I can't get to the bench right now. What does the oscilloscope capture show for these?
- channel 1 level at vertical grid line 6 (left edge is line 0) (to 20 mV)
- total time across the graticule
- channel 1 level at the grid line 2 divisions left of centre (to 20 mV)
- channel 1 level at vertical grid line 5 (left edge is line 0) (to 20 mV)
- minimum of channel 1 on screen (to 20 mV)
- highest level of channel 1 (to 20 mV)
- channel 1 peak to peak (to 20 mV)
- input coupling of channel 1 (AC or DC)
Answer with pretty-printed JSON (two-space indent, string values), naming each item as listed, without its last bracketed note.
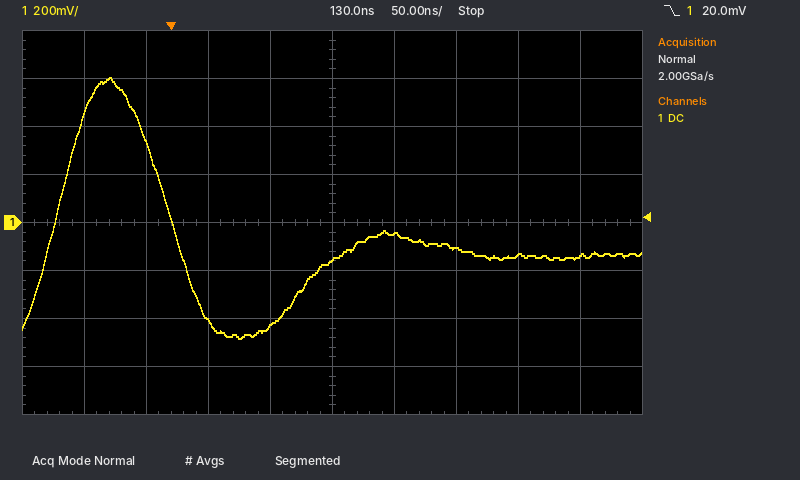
{
  "channel 1 level at vertical grid line 6 (left edge is line 0)": "-40 mV",
  "total time across the graticule": "500 ns",
  "channel 1 level at the grid line 2 divisions left of centre": "-400 mV",
  "channel 1 level at vertical grid line 5 (left edge is line 0)": "-160 mV",
  "minimum of channel 1 on screen": "-480 mV",
  "highest level of channel 1": "600 mV",
  "channel 1 peak to peak": "1.08 V",
  "input coupling of channel 1": "DC"
}
